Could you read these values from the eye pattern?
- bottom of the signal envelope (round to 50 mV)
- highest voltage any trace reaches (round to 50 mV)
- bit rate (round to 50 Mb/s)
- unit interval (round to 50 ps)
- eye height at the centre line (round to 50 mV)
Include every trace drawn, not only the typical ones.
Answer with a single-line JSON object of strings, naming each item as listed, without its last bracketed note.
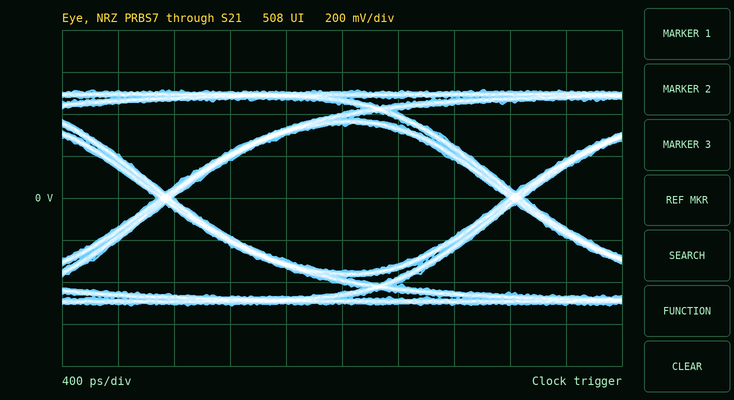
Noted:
{"bottom of the signal envelope": "-500 mV", "highest voltage any trace reaches": "500 mV", "bit rate": "400 Mb/s", "unit interval": "2.50 ns", "eye height at the centre line": "700 mV"}
